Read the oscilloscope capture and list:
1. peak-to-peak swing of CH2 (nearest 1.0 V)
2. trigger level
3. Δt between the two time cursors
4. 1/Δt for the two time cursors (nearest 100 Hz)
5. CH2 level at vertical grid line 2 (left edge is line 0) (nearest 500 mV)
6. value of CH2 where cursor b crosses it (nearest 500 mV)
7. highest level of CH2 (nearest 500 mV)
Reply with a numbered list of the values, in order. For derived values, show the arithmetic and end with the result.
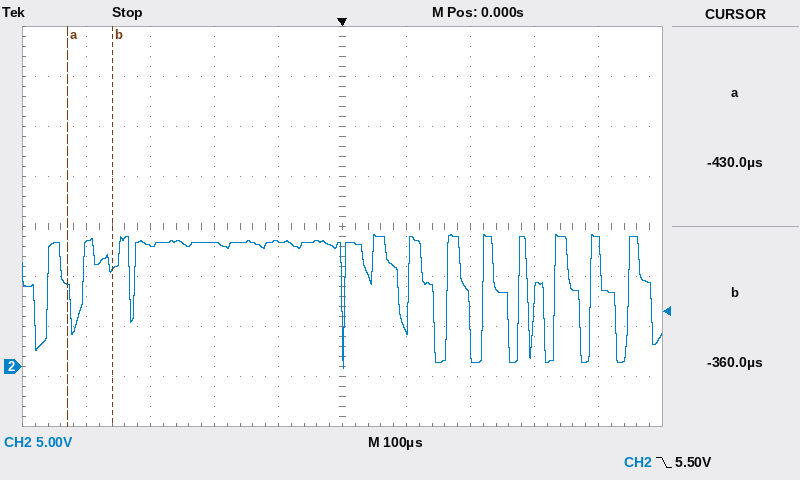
1. 13.0 V
2. 5.50 V
3. -360 µs − (-430 µs) = 70 µs
4. 1 / 70 µs ≈ 14.3 kHz
5. 12.0 V
6. 10.0 V
7. 13.0 V
